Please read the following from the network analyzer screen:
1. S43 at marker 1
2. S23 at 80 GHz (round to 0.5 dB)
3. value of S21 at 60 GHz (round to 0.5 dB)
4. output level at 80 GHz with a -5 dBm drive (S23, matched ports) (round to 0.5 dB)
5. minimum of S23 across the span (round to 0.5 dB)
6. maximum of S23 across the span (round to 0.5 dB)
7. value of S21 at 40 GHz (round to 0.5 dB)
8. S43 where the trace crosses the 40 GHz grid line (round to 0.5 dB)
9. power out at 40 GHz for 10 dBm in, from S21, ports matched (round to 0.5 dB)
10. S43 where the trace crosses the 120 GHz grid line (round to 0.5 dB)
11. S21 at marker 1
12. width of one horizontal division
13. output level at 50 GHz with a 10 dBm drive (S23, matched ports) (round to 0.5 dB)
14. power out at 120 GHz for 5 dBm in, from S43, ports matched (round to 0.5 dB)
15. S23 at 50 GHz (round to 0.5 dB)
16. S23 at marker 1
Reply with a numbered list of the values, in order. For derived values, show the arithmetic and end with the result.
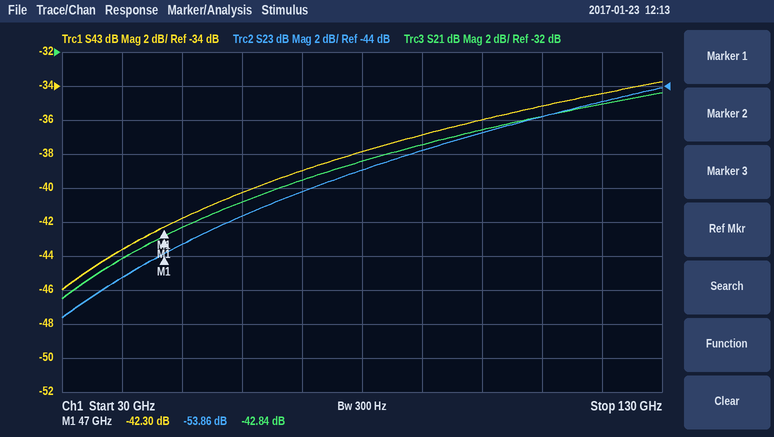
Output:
1. -42.30 dB
2. -49.0 dB
3. -41.0 dB
4. -5 dBm + (-49.0 dB) = -54.0 dBm
5. -57.5 dB
6. -44.0 dB
7. -44.0 dB
8. -43.5 dB
9. 10 dBm + (-44.0 dB) = -34.0 dBm
10. -34.5 dB
11. -42.84 dB
12. 10 GHz
13. 10 dBm + (-53.5 dB) = -43.5 dBm
14. 5 dBm + (-34.5 dB) = -29.5 dBm
15. -53.5 dB
16. -53.86 dB
